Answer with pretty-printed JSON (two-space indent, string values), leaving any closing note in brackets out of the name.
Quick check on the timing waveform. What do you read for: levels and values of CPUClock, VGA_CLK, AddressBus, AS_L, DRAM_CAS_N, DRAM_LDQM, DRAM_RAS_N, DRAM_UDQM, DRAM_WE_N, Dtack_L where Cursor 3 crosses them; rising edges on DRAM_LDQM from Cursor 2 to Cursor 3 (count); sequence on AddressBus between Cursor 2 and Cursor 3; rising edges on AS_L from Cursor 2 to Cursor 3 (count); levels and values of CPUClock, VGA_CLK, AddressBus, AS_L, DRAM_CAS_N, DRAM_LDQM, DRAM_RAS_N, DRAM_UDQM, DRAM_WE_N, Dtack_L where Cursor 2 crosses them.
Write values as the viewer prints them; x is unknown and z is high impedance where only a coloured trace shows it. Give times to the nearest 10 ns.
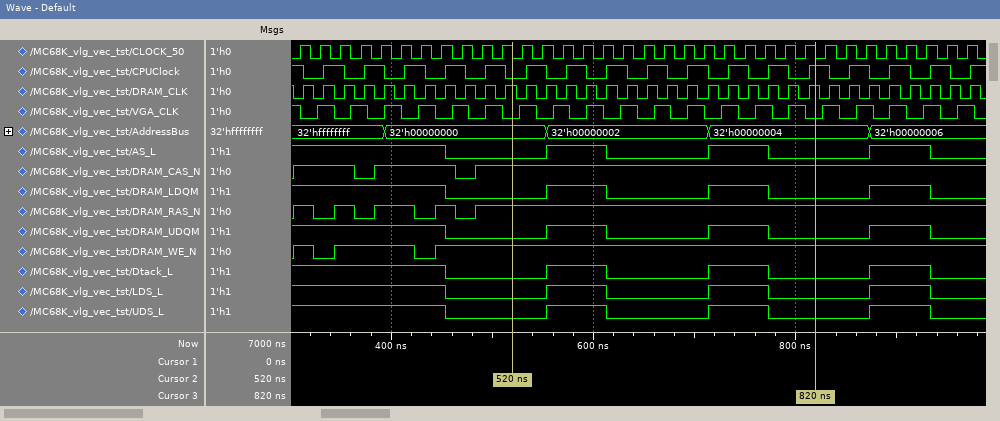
{
  "levels and values of CPUClock, VGA_CLK, AddressBus, AS_L, DRAM_CAS_N, DRAM_LDQM, DRAM_RAS_N, DRAM_UDQM, DRAM_WE_N, Dtack_L where Cursor 3 crosses them": "CPUClock=1, VGA_CLK=0, AddressBus=32'h00000004, AS_L=0, DRAM_CAS_N=1, DRAM_LDQM=0, DRAM_RAS_N=1, DRAM_UDQM=0, DRAM_WE_N=1, Dtack_L=0",
  "rising edges on DRAM_LDQM from Cursor 2 to Cursor 3": "2",
  "sequence on AddressBus between Cursor 2 and Cursor 3": "32'h00000000, 32'h00000002, 32'h00000004",
  "rising edges on AS_L from Cursor 2 to Cursor 3": "2",
  "levels and values of CPUClock, VGA_CLK, AddressBus, AS_L, DRAM_CAS_N, DRAM_LDQM, DRAM_RAS_N, DRAM_UDQM, DRAM_WE_N, Dtack_L where Cursor 2 crosses them": "CPUClock=0, VGA_CLK=0, AddressBus=32'h00000000, AS_L=0, DRAM_CAS_N=1, DRAM_LDQM=0, DRAM_RAS_N=1, DRAM_UDQM=0, DRAM_WE_N=1, Dtack_L=0"
}
